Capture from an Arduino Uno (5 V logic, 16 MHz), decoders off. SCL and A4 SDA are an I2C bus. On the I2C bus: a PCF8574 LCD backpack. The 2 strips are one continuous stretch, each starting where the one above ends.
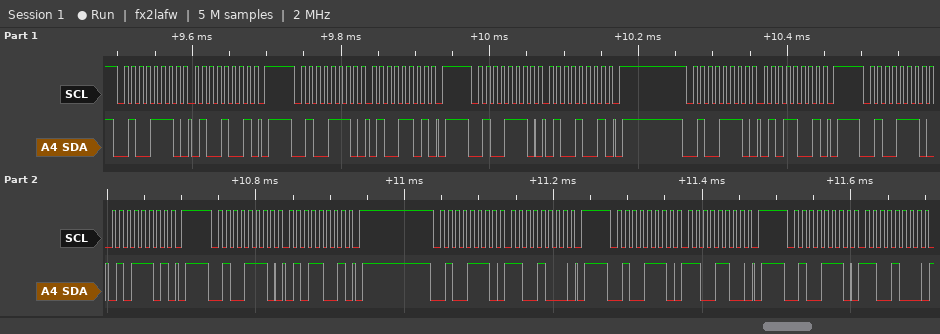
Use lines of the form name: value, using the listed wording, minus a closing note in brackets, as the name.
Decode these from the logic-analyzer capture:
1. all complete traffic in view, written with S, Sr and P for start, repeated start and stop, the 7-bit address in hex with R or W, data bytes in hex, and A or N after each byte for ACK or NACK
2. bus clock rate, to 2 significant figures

all complete traffic in view, written with S, Sr and P for start, repeated start and stop, the 7-bit address in hex with R or W, data bytes in hex, and A or N after each byte for ACK or NACK: S 27W A 49 A P S 27W A 4D A P S 27W A 49 A P S 27W A 59 A P S 27W A 5D A P S 27W A 59 A P S 27W A C8 A P S 27W A CC A P S 27W A C8 A
bus clock rate, to 2 significant figures: 100 kHz
